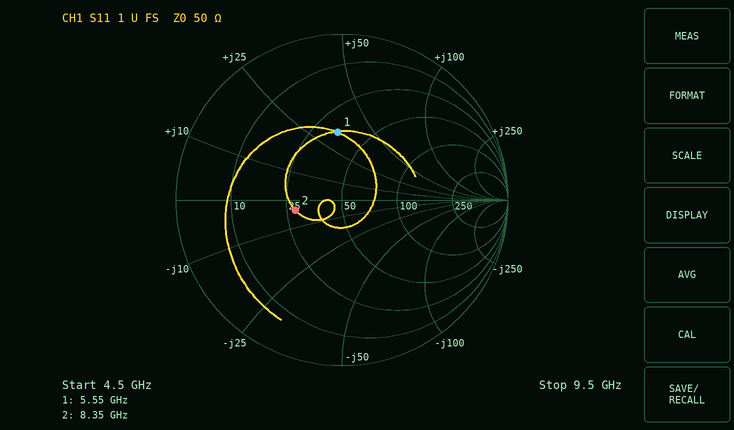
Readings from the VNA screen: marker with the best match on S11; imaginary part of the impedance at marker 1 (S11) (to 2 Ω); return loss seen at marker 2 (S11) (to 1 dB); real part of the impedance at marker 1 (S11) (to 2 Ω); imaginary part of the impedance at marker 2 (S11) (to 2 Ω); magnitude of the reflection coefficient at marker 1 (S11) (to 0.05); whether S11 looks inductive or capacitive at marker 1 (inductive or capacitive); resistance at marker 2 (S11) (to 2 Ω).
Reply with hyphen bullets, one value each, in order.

- marker 2
- +34 Ω
- 11 dB
- 34 Ω
- -4 Ω
- 0.40
- inductive
- 28 Ω
